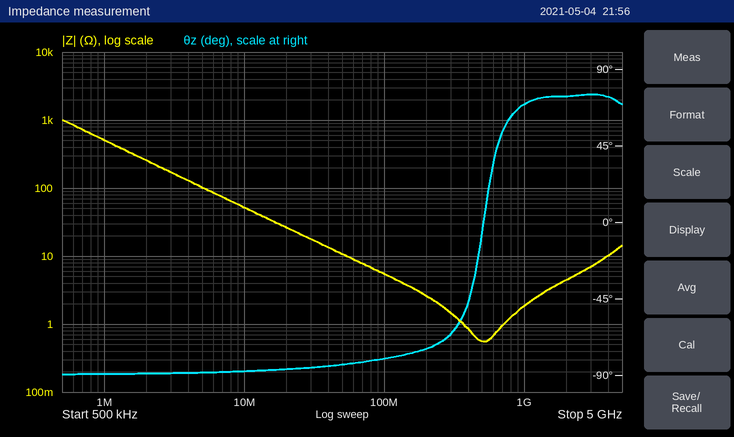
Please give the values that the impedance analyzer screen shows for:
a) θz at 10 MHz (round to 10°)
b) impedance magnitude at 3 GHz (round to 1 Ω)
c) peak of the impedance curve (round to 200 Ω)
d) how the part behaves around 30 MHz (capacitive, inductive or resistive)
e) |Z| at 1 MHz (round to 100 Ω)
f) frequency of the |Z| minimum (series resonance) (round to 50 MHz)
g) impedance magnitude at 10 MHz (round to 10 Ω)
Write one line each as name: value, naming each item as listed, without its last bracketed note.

θz at 10 MHz: -90°
impedance magnitude at 3 GHz: 7 Ω
peak of the impedance curve: 1.0 kΩ
how the part behaves around 30 MHz: capacitive
|Z| at 1 MHz: 500 Ω
frequency of the |Z| minimum (series resonance): 500 MHz
impedance magnitude at 10 MHz: 50 Ω
